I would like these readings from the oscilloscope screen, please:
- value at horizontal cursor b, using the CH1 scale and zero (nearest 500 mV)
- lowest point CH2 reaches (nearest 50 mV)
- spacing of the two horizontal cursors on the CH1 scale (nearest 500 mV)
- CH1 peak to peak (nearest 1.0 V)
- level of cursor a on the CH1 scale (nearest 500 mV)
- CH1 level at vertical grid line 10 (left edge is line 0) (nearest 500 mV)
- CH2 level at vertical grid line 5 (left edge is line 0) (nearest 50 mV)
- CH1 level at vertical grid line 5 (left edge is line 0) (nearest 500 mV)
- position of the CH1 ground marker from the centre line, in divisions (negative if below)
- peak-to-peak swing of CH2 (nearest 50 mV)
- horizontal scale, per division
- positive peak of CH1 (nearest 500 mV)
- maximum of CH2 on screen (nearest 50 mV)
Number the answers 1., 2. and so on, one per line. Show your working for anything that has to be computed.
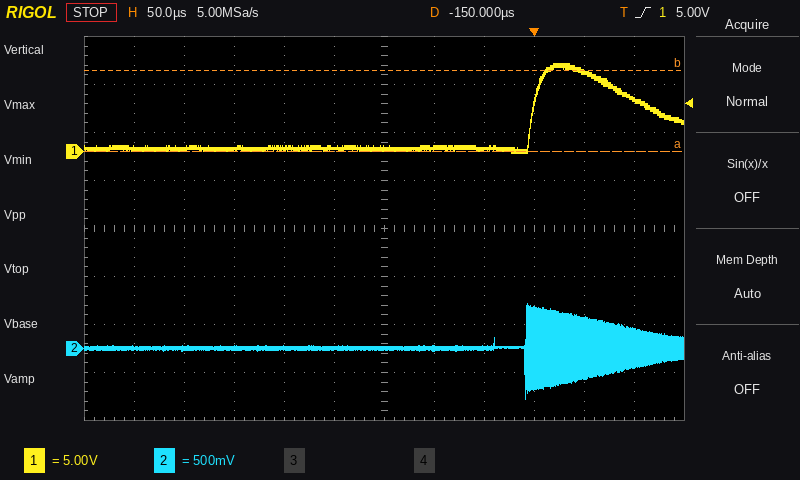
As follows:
1. 8.5 V
2. -550 mV
3. 8.5 V
4. 9.0 V
5. 0.0 V
6. 8.5 V
7. 0 mV
8. 500 mV
9. +1.6 div
10. 450 mV − (-550 mV) = 1.00 V
11. 50 µs
12. 9.0 V
13. 450 mV
